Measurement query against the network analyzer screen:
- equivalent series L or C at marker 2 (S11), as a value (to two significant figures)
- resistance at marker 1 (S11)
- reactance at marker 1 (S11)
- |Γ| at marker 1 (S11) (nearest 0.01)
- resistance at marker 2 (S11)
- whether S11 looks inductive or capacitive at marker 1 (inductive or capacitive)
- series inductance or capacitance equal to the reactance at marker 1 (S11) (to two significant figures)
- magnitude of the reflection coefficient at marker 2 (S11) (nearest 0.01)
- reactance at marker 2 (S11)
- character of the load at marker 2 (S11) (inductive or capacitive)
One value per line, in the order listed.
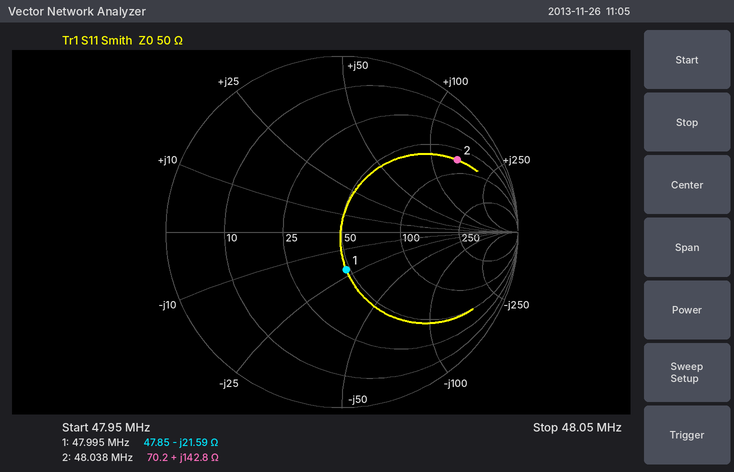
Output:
470 nH
47.85 Ω
-21.59 Ω
0.22
70.2 Ω
capacitive
150 pF
0.77
+142.8 Ω
inductive
